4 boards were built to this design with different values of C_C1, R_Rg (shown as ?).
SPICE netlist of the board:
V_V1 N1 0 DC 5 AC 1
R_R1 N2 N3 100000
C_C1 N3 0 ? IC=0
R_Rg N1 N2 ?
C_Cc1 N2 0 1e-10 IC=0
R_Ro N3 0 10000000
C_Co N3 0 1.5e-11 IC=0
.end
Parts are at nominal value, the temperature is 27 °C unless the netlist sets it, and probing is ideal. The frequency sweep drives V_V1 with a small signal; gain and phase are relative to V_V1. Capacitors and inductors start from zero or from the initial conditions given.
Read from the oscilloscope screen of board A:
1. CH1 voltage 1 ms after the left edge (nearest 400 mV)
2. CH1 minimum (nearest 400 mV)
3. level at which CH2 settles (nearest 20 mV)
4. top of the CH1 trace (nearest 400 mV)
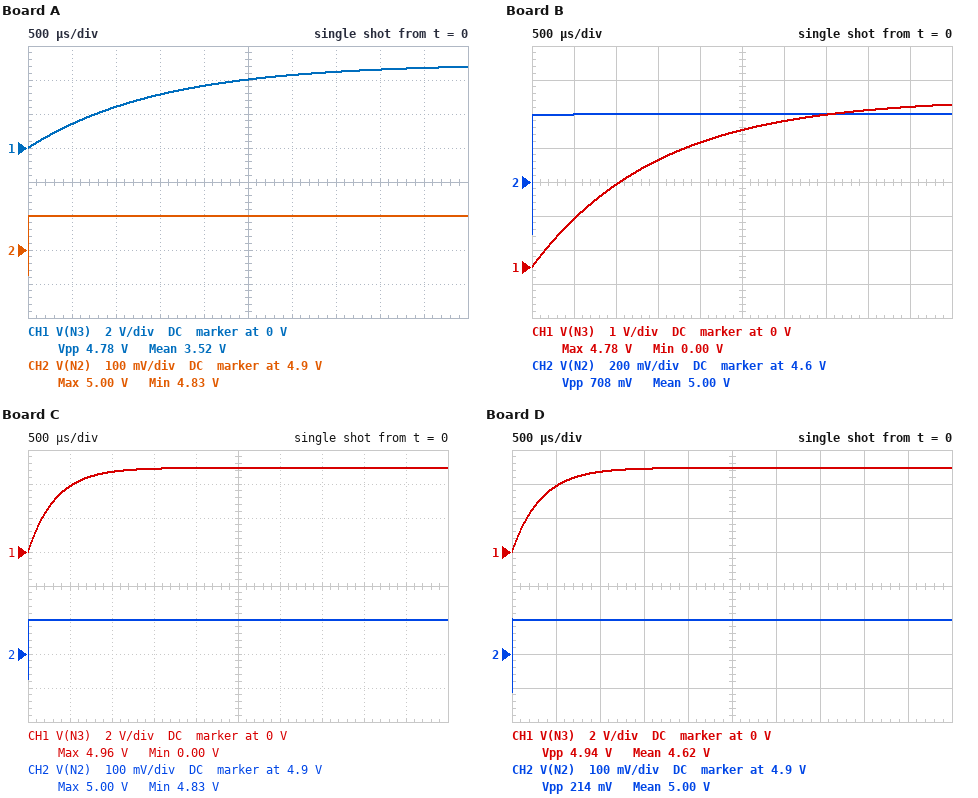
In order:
2.4 V
0 V
5.00 V
4.8 V
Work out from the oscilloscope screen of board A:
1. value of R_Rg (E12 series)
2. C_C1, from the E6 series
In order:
18 Ω
15 nF
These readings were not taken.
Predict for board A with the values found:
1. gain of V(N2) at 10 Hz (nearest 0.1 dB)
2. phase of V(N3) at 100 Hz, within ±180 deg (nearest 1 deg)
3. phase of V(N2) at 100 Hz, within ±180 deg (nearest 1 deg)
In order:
0 dB
-43 deg
0 deg
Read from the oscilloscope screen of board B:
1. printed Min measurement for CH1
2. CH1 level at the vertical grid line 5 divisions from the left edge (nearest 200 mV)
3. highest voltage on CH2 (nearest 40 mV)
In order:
0.00 V
4.0 V
5.00 V
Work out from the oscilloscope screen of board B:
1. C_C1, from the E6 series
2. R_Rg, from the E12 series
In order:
15 nF
82 Ω
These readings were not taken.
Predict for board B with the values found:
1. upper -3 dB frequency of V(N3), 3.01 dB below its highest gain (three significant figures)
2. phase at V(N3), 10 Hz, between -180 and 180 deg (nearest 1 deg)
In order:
107 Hz
-5 deg
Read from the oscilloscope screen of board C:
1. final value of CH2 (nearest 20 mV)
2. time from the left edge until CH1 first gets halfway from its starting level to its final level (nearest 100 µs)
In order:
5.00 V
200 µs
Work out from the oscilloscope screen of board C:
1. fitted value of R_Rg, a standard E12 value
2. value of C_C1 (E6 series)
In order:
18 Ω
3.3 nF
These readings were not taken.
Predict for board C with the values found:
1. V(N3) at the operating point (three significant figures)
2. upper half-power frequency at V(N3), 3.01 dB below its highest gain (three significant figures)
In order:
4.95 V
485 Hz
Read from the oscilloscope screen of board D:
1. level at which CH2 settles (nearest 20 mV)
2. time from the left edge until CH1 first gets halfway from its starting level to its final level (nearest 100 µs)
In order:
5.00 V
200 µs
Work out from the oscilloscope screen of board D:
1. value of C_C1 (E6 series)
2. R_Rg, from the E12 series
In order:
3.3 nF
22 Ω
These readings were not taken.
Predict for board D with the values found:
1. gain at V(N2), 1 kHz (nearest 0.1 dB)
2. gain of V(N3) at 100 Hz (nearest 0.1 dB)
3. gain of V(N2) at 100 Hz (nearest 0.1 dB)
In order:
0 dB
-0.3 dB
0 dB
